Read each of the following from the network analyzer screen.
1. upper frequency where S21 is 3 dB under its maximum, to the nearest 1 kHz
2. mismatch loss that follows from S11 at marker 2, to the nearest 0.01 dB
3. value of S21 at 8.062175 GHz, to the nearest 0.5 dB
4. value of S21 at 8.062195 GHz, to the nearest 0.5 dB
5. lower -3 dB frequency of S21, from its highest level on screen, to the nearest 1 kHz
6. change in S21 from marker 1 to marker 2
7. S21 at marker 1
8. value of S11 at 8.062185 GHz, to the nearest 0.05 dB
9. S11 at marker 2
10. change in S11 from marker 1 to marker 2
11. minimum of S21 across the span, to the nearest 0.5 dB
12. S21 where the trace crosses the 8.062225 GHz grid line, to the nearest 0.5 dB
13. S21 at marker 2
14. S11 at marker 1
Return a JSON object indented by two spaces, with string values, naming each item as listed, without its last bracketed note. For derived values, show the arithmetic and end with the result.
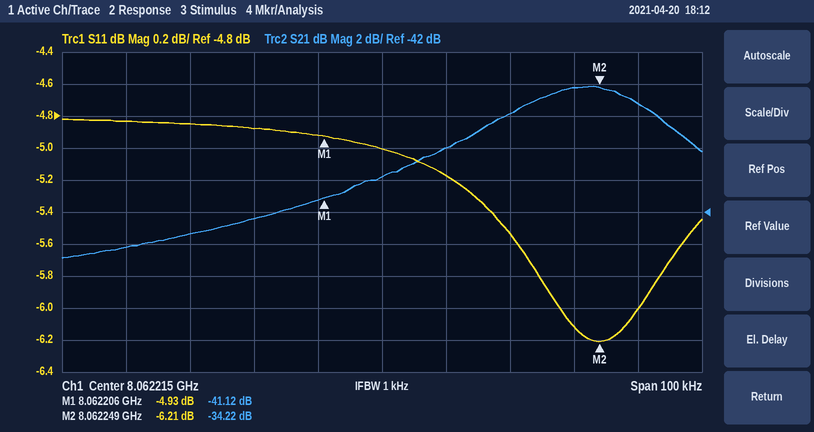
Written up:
{
  "upper frequency where S21 is 3 dB under its maximum, to the nearest 1 kHz": "8.062262 GHz",
  "mismatch loss that follows from S11 at marker 2, to the nearest 0.01 dB": "−10 log10(1 − 10^(-6.21/10)) ≈ 1.19 dB",
  "value of S21 at 8.062175 GHz, to the nearest 0.5 dB": "-44.0 dB",
  "value of S21 at 8.062195 GHz, to the nearest 0.5 dB": "-42.5 dB",
  "lower -3 dB frequency of S21, from its highest level on screen, to the nearest 1 kHz": "8.062229 GHz",
  "change in S21 from marker 1 to marker 2": "-34.22 − (-41.12) = 6.90 dB",
  "S21 at marker 1": "-41.12 dB",
  "value of S11 at 8.062185 GHz, to the nearest 0.05 dB": "-4.85 dB",
  "S11 at marker 2": "-6.21 dB",
  "change in S11 from marker 1 to marker 2": "-6.21 − (-4.93) = -1.28 dB",
  "minimum of S21 across the span, to the nearest 0.5 dB": "-45.0 dB",
  "S21 where the trace crosses the 8.062225 GHz grid line, to the nearest 0.5 dB": "-38.0 dB",
  "S21 at marker 2": "-34.22 dB",
  "S11 at marker 1": "-4.93 dB"
}
